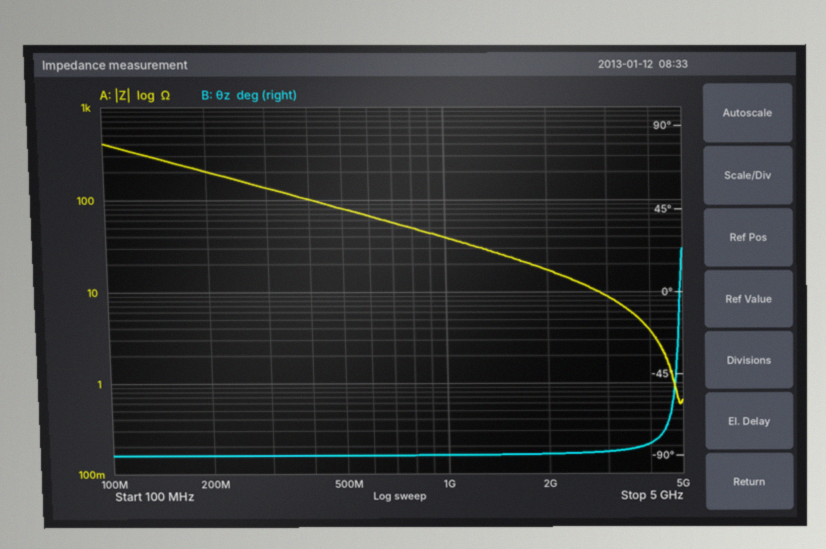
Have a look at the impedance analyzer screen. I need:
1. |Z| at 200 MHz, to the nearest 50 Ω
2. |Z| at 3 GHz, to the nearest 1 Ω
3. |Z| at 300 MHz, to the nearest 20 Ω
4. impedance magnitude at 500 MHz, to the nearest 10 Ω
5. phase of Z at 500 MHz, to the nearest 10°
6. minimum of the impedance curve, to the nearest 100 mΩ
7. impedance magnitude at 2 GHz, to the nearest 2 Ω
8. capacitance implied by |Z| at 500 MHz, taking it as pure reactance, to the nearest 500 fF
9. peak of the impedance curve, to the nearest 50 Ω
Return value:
200 Ω
9 Ω
140 Ω
80 Ω
-90°
600 mΩ
18 Ω
4.0 pF
400 Ω
